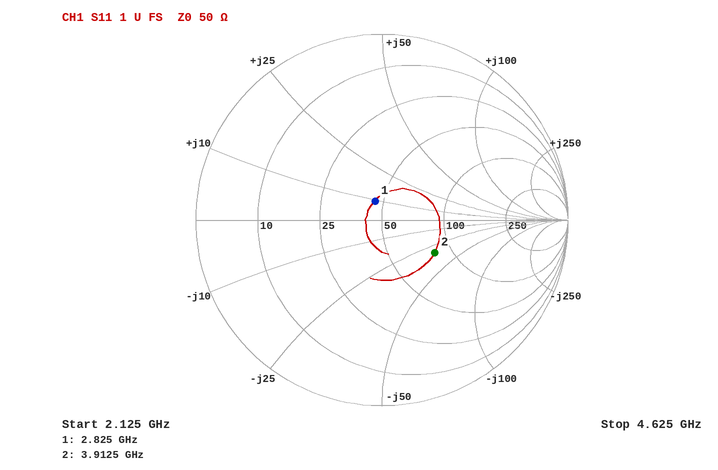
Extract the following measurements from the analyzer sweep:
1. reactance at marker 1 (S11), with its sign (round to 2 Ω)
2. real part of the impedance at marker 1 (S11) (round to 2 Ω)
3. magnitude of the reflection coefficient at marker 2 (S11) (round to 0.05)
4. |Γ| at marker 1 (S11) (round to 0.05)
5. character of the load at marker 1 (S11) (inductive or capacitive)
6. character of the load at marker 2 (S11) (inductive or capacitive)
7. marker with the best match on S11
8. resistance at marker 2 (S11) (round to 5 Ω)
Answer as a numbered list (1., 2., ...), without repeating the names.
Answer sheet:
1. +10 Ω
2. 46 Ω
3. 0.35
4. 0.10
5. inductive
6. capacitive
7. marker 1
8. 80 Ω
